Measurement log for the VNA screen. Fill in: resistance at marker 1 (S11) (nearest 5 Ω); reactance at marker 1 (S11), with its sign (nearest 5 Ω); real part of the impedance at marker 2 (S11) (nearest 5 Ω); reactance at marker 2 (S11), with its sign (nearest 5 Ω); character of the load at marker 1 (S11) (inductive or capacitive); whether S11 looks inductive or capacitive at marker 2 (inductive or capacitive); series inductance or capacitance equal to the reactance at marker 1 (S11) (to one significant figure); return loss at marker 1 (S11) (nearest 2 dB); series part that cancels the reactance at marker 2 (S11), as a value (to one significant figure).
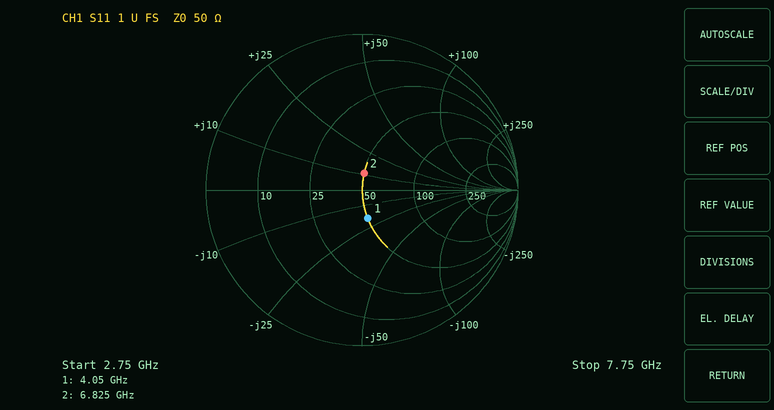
50 Ω
-20 Ω
50 Ω
+10 Ω
capacitive
inductive
2 pF
14 dB
2 pF
